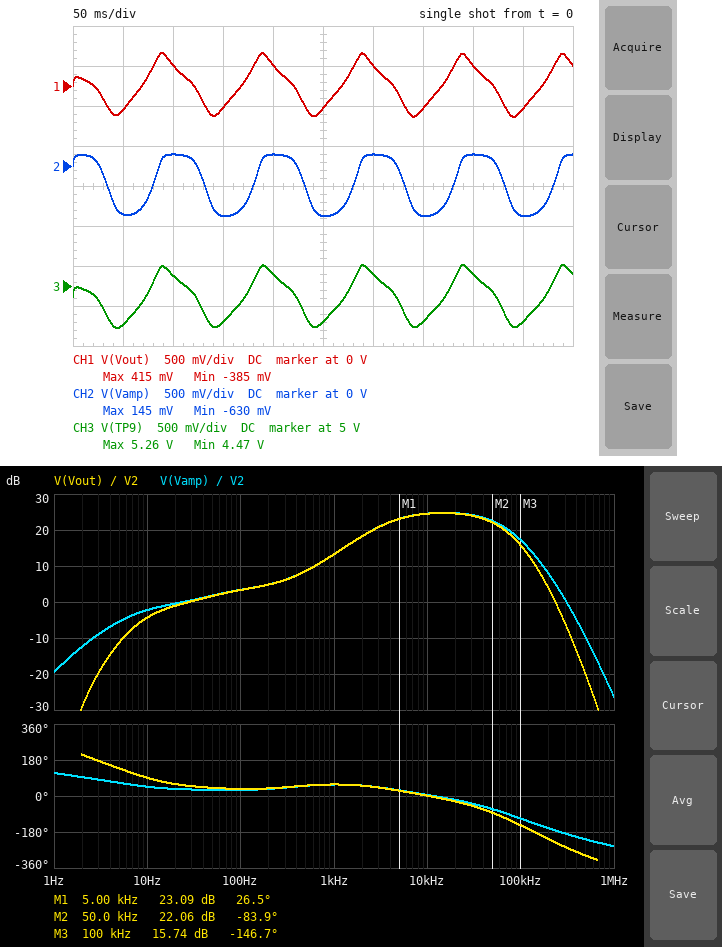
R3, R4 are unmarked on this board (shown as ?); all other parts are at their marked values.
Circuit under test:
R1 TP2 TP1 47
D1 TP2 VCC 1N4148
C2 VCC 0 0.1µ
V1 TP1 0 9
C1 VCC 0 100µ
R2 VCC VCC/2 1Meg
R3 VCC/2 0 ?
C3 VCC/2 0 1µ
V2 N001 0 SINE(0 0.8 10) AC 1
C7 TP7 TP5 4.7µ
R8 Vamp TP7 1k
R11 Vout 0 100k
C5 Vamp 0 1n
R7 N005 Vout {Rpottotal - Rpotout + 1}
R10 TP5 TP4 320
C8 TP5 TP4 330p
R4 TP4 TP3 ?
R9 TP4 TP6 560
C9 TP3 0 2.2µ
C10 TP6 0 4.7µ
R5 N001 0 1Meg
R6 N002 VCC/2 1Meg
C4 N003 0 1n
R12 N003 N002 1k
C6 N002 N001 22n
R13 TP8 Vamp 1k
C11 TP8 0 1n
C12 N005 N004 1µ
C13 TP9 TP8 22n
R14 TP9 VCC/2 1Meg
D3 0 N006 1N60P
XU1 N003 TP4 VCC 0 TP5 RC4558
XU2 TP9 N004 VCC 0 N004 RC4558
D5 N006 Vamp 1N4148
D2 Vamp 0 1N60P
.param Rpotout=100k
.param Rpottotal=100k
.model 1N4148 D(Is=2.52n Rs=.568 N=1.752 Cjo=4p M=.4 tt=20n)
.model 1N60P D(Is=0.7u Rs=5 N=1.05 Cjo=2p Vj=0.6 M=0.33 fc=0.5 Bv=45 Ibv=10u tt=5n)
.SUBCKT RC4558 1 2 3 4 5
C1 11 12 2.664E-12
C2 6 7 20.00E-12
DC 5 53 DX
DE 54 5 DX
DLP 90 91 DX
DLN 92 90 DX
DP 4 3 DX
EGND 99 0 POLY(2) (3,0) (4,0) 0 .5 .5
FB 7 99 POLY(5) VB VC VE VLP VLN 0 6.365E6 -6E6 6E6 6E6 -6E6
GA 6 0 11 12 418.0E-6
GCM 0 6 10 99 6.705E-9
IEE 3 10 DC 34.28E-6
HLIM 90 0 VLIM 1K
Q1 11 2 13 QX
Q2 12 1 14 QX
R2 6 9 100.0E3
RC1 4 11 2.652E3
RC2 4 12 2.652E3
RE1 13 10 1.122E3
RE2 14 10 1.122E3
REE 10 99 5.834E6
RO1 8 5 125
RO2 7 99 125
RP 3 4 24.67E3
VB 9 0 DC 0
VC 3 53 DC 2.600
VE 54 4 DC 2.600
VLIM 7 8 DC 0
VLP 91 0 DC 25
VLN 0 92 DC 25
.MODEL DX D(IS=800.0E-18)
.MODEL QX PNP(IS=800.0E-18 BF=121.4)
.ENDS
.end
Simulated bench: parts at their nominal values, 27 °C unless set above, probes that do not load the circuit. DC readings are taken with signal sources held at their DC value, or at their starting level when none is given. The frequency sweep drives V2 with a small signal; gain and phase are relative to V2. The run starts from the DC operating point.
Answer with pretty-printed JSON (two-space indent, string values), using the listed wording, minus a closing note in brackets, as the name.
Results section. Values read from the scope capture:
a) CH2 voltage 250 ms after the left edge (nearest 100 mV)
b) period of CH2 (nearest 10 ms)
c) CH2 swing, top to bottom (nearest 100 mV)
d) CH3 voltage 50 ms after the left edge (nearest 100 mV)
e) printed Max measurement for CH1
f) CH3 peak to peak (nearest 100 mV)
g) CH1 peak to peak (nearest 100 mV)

{
  "CH2 voltage 250 ms after the left edge": "-600 mV",
  "period of CH2": "100 ms",
  "CH2 swing, top to bottom": "800 mV",
  "CH3 voltage 50 ms after the left edge": "4.5 V",
  "printed Max measurement for CH1": "415 mV",
  "CH3 peak to peak": "800 mV",
  "CH1 peak to peak": "800 mV"
}
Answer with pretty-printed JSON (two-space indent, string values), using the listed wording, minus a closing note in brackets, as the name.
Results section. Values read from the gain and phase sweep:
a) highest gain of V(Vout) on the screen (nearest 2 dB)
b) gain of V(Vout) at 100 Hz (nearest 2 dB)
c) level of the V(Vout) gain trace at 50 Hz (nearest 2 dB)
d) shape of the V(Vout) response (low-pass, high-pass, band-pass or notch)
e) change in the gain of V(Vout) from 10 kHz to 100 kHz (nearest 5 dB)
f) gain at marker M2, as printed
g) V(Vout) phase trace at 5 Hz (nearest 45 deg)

{
  "highest gain of V(Vout) on the screen": "24 dB",
  "gain of V(Vout) at 100 Hz": "4 dB",
  "level of the V(Vout) gain trace at 50 Hz": "2 dB",
  "shape of the V(Vout) response": "band-pass",
  "change in the gain of V(Vout) from 10 kHz to 100 kHz": "-10 dB",
  "gain at marker M2, as printed": "22.06 dB",
  "V(Vout) phase trace at 5 Hz": "135 deg"
}
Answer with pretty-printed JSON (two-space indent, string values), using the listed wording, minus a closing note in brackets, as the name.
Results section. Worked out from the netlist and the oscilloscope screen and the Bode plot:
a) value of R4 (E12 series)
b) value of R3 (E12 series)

{
  "value of R4": "18 Ω",
  "value of R3": "1.2 MΩ"
}
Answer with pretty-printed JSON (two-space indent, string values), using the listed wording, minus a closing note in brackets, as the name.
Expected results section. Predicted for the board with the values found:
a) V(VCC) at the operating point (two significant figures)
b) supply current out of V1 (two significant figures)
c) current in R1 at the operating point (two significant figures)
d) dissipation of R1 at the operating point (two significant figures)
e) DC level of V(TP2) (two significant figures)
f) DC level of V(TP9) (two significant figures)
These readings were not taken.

{
  "V(VCC) at the operating point": "8.4 V",
  "supply current out of V1": "750 µA",
  "current in R1 at the operating point": "750 µA",
  "dissipation of R1 at the operating point": "27 µW",
  "DC level of V(TP2)": "9.0 V",
  "DC level of V(TP9)": "4.9 V"
}
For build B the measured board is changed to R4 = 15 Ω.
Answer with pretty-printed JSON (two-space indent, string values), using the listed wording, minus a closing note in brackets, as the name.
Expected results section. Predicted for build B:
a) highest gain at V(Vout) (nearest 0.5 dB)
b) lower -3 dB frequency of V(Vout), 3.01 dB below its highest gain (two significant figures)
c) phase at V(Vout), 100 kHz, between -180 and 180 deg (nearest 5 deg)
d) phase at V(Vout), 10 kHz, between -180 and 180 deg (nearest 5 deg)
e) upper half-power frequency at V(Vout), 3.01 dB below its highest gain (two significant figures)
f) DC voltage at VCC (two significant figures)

{
  "highest gain at V(Vout)": "26.0 dB",
  "lower -3 dB frequency of V(Vout), 3.01 dB below its highest gain": "4.2 kHz",
  "phase at V(Vout), 100 kHz, between -180 and 180 deg": "-150 deg",
  "phase at V(Vout), 10 kHz, between -180 and 180 deg": "5 deg",
  "upper half-power frequency at V(Vout), 3.01 dB below its highest gain": "52 kHz",
  "DC voltage at VCC": "8.4 V"
}
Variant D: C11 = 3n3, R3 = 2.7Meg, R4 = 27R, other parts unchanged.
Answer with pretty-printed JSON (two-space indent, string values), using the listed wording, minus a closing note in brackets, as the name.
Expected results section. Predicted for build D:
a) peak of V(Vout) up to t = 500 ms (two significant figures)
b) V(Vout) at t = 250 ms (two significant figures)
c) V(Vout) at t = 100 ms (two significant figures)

{
  "peak of V(Vout) up to t = 500 ms": "130 mV",
  "V(Vout) at t = 250 ms": "-270 mV",
  "V(Vout) at t = 100 ms": "79 mV"
}
